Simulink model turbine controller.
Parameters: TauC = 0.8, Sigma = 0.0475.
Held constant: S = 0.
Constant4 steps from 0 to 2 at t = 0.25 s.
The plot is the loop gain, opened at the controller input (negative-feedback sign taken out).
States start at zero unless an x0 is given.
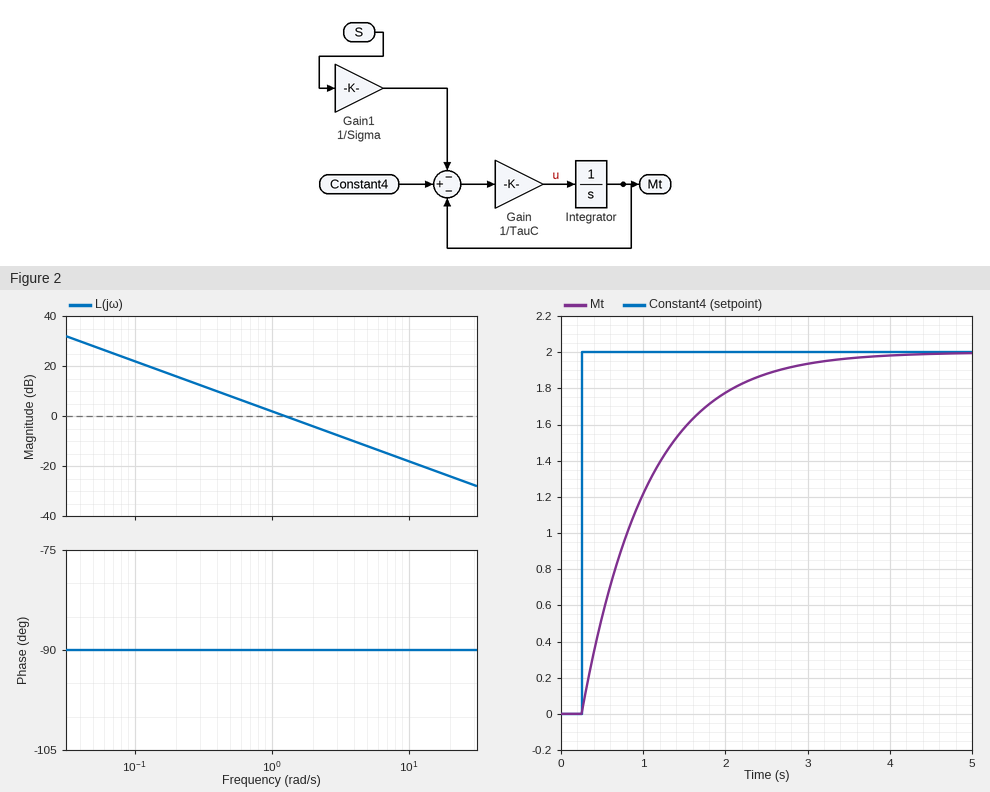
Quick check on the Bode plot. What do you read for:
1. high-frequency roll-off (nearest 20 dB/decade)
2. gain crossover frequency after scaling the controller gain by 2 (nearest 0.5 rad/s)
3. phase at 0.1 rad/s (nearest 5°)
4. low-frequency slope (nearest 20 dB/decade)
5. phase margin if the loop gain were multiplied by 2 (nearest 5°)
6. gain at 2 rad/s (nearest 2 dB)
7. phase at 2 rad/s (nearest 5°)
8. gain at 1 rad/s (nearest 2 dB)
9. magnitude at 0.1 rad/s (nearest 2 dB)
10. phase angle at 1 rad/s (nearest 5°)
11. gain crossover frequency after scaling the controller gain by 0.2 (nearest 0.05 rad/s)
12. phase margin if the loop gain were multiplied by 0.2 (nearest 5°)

-20 dB/decade
2.5 rad/s
-90°
-20 dB/decade
90°
-4 dB
-90°
2 dB
22 dB
-90°
0.25 rad/s
90°
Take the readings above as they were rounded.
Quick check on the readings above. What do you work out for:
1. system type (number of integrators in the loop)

1
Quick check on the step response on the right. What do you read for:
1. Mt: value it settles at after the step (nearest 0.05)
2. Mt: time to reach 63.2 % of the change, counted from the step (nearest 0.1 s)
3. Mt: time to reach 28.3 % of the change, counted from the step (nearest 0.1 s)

2.00
0.8 s
0.3 s
